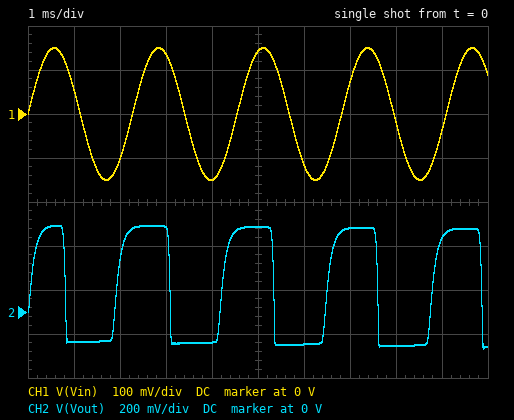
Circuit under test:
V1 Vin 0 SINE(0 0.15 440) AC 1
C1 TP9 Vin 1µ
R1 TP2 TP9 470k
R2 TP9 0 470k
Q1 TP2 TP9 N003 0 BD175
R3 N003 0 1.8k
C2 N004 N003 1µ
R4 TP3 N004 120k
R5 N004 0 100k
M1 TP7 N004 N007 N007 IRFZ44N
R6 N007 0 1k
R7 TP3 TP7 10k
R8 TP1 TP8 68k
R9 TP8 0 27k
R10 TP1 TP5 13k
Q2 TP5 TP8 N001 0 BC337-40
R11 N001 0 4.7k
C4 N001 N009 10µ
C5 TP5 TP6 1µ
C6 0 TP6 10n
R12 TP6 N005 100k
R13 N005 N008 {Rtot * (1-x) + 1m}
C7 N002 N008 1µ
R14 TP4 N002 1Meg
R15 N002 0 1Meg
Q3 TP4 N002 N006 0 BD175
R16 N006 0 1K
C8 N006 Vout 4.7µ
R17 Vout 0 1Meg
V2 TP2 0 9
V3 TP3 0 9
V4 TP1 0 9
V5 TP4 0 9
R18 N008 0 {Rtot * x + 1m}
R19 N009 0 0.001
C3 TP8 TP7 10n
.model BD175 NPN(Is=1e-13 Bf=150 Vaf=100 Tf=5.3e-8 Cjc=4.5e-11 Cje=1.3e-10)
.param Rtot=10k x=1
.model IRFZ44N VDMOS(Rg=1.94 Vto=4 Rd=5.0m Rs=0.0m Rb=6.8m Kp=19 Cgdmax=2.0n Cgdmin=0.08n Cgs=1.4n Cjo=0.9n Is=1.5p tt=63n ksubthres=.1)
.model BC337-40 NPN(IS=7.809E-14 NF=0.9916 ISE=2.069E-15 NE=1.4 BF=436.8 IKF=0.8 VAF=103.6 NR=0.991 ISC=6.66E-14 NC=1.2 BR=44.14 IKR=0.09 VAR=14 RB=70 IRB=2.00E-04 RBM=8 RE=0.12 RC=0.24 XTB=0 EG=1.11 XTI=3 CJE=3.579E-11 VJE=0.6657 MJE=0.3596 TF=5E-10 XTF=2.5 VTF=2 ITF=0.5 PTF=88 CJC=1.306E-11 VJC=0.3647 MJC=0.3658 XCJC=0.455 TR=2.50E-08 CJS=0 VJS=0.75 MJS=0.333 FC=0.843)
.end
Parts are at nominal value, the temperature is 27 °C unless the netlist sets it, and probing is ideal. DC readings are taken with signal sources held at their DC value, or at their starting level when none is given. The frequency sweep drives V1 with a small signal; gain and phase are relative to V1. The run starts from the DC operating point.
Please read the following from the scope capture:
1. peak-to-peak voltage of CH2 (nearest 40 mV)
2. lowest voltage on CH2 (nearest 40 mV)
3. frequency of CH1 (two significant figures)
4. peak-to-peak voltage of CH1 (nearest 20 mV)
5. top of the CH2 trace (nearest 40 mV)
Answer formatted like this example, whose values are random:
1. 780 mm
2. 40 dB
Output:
1. 560 mV
2. -160 mV
3. 440 Hz
4. 300 mV
5. 400 mV
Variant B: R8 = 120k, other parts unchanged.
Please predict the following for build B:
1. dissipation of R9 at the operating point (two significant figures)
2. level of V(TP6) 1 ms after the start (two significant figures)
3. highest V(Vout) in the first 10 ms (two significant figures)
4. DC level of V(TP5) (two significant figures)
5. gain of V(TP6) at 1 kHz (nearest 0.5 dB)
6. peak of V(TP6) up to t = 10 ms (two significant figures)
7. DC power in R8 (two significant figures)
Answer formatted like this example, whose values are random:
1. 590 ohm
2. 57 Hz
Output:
1. 100 µW
2. -4.9 V
3. 230 mV
4. 6.0 V
5. 50.5 dB
6. 2.7 V
7. 450 µW
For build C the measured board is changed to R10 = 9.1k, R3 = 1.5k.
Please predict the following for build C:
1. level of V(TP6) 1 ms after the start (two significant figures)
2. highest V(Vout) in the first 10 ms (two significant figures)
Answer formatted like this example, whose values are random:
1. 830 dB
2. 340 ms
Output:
1. -3.2 V
2. 290 mV
